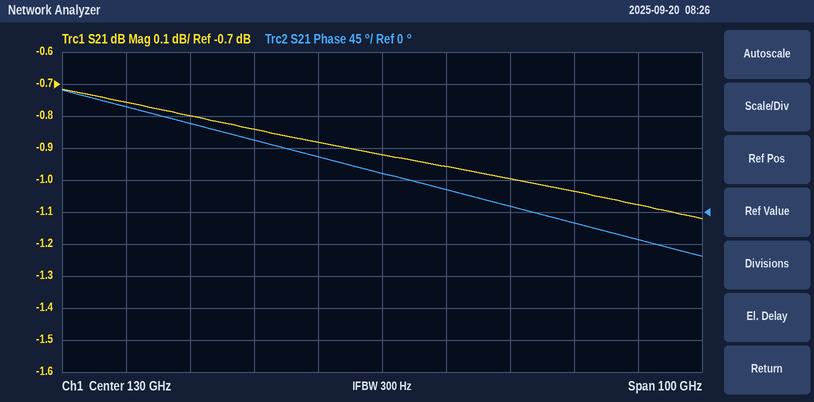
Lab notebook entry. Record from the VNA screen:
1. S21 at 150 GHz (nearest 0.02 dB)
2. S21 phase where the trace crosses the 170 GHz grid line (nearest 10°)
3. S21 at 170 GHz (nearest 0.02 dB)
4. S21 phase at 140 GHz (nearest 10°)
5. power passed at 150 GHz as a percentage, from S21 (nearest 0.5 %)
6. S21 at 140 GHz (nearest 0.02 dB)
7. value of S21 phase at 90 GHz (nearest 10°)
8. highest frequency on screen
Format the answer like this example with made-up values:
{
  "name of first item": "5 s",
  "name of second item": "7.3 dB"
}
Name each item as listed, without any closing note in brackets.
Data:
{
  "S21 at 150 GHz": "-1.00 dB",
  "S21 phase where the trace crosses the 170 GHz grid line": "-40°",
  "S21 at 170 GHz": "-1.08 dB",
  "S21 phase at 140 GHz": "30°",
  "power passed at 150 GHz as a percentage, from S21": "79.5 %",
  "S21 at 140 GHz": "-0.96 dB",
  "value of S21 phase at 90 GHz": "150°",
  "highest frequency on screen": "180 GHz"
}
